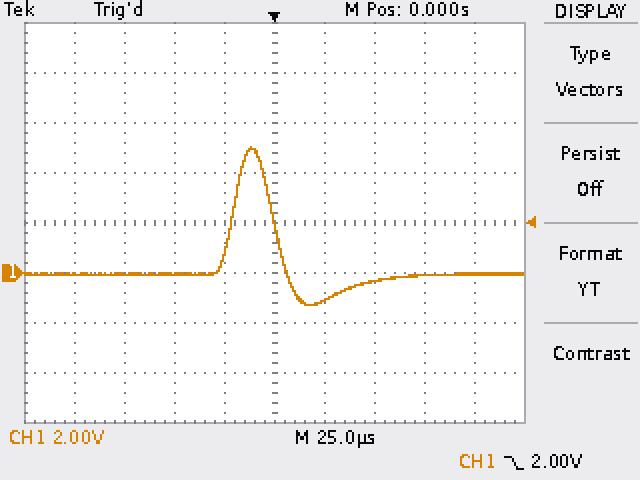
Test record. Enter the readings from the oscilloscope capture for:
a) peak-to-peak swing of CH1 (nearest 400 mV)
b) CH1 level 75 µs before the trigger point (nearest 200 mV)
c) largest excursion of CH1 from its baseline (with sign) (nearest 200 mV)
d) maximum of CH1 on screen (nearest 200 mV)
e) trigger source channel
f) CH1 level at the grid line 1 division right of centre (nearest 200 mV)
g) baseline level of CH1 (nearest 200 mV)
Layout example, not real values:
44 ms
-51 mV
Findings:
6.4 V
0.0 V
+5.0 V
5.0 V
CH1
-1.2 V
0.0 V
